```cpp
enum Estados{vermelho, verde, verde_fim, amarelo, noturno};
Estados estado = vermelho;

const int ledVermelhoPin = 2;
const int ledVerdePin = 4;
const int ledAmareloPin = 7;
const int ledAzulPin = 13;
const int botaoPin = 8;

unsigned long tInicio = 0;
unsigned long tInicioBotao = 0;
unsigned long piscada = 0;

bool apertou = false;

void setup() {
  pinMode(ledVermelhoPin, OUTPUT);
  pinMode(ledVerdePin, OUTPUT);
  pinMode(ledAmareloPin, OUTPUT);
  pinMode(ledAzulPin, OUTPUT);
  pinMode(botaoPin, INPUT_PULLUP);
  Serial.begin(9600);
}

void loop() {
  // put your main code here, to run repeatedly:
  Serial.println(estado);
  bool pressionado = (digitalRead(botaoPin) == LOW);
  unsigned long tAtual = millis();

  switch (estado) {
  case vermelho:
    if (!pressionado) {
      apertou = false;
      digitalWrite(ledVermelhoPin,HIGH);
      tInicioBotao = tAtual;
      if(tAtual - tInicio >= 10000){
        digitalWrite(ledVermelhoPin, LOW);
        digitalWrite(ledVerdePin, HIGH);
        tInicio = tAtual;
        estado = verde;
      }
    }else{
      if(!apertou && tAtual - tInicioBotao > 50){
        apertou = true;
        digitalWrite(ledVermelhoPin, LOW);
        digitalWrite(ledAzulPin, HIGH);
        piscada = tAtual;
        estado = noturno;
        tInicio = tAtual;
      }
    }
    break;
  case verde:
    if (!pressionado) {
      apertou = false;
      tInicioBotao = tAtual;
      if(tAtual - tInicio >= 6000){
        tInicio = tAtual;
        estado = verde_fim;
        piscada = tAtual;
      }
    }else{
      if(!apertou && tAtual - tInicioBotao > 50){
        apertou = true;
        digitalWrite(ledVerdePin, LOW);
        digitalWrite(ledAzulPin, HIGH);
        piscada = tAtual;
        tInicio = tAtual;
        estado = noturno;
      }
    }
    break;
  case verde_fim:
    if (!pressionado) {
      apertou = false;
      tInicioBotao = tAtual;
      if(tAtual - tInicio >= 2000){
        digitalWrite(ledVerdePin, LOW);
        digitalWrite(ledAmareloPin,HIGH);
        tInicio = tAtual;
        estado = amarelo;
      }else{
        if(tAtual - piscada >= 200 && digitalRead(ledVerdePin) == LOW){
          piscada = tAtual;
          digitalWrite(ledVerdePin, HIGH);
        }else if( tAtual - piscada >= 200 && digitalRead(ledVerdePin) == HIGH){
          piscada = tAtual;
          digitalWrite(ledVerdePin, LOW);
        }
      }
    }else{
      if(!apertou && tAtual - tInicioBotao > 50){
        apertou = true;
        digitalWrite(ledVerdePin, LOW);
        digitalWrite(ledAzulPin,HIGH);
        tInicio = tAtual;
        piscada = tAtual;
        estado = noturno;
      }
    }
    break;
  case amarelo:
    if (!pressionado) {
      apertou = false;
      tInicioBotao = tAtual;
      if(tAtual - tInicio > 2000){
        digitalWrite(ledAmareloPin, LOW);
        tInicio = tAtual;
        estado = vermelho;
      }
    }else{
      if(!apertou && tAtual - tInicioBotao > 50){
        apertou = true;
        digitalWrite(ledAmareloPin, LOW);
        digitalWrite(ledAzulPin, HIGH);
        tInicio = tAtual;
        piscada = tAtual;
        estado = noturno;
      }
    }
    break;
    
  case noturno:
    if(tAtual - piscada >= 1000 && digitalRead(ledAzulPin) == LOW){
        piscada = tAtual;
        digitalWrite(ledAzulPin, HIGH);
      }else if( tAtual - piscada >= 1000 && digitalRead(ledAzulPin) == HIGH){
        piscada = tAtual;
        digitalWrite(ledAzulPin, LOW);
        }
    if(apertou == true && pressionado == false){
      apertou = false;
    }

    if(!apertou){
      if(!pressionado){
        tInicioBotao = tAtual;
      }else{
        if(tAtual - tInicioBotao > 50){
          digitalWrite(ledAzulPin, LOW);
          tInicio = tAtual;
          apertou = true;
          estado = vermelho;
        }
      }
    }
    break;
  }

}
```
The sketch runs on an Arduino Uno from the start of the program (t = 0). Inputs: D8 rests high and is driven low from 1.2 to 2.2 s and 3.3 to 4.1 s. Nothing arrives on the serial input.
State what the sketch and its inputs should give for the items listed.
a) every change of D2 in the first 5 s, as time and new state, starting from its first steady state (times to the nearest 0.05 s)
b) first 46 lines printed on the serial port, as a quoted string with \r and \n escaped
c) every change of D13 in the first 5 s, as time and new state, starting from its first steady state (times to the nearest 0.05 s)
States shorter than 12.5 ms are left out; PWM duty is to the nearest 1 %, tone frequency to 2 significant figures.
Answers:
0 s high; 1.25 s low; 4.1 s high
"0\r\n0\r\n0\r\n0\r\n0\r\n0\r\n0\r\n0\r\n0\r\n0\r\n0\r\n0\r\n0\r\n0\r\n0\r\n0\r\n0\r\n0\r\n0\r\n0\r\n0\r\n0\r\n0\r\n0\r\n0\r\n0\r\n0\r\n0\r\n0\r\n0\r\n0\r\n0\r\n0\r\n0\r\n0\r\n0\r\n0\r\n0\r\n0\r\n0\r\n0\r\n0\r\n0\r\n0\r\n0\r\n0\r\n"
0 s low; 1.25 s high; 2.25 s low; 3.25 s high; 3.35 s low
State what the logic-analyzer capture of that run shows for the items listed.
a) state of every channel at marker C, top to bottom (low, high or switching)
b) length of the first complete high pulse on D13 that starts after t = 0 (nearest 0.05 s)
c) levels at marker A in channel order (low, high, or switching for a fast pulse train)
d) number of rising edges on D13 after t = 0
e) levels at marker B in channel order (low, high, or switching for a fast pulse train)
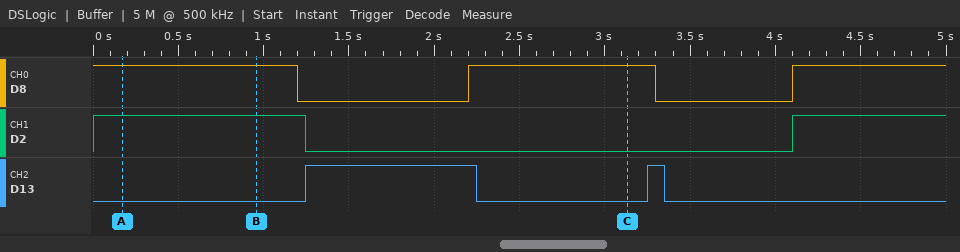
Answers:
D8 high, D2 low, D13 low
1.00 s
D8 high, D2 high, D13 low
2
D8 high, D2 high, D13 low
